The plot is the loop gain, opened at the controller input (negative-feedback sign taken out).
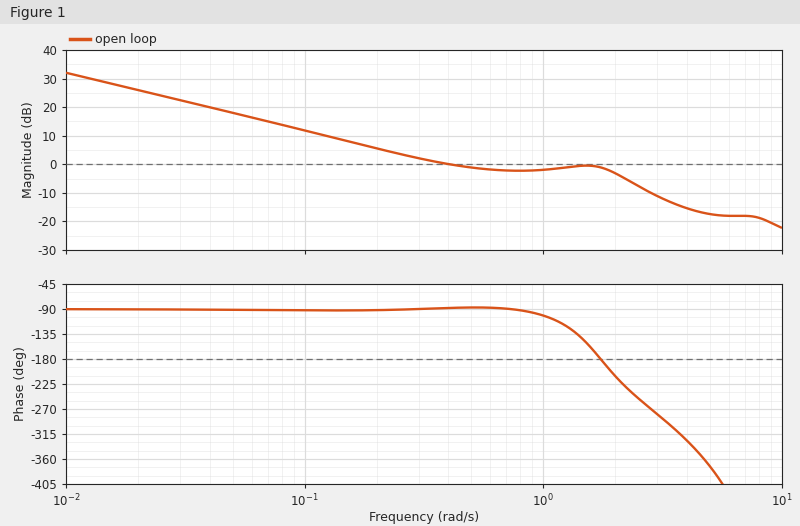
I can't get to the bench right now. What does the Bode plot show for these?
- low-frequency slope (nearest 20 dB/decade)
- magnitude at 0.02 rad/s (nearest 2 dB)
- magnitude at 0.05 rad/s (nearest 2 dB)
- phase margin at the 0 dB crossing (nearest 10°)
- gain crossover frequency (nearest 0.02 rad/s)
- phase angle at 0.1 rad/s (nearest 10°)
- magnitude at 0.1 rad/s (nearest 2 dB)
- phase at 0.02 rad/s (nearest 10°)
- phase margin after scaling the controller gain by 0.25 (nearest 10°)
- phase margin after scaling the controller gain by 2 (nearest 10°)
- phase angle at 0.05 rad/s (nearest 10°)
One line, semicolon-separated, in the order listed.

-20 dB/decade; 26 dB; 18 dB; 90°; 0.40 rad/s; -90°; 12 dB; -90°; 90°; -60°; -90°
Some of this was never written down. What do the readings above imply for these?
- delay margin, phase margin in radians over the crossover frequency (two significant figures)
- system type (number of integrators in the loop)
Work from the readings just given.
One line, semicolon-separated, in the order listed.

3.9 s; 1
